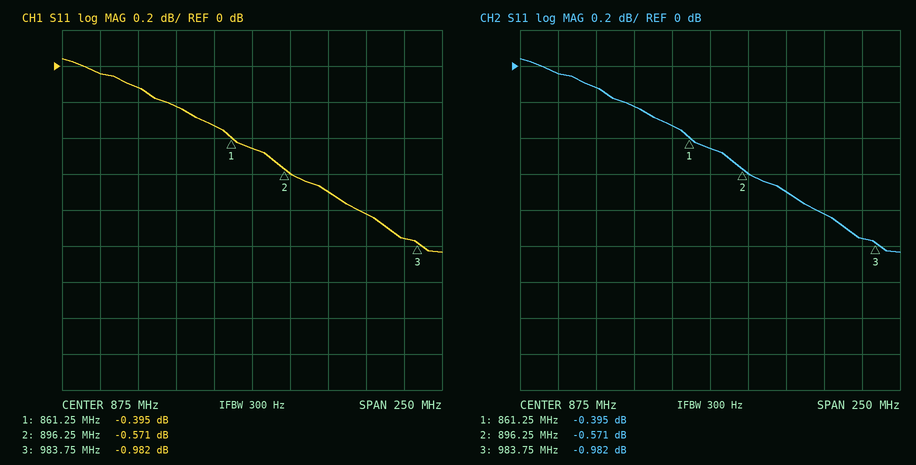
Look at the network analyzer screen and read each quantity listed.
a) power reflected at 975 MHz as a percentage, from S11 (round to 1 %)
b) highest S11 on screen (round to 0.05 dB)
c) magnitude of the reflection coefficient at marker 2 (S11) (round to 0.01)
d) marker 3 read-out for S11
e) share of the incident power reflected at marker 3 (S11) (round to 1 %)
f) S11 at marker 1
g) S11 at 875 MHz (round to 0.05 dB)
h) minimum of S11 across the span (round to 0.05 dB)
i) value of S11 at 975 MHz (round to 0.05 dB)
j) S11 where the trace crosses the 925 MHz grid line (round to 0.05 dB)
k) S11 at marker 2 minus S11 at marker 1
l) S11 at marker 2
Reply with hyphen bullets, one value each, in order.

- 80 %
- 0.05 dB
- 0.94
- -0.982 dB
- 80 %
- -0.395 dB
- -0.45 dB
- -1.05 dB
- -0.95 dB
- -0.70 dB
- -0.176 dB
- -0.571 dB
